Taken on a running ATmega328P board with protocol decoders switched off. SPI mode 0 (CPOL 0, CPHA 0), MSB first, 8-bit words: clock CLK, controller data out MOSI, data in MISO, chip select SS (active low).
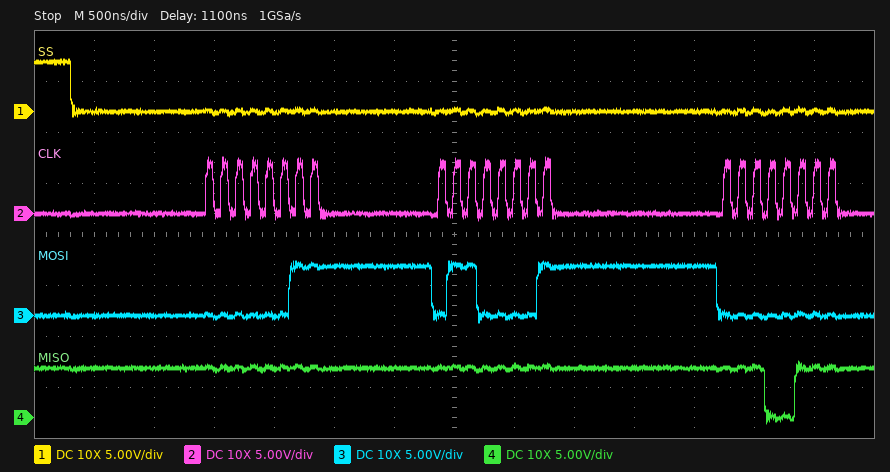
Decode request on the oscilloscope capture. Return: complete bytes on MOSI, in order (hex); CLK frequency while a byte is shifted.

03 61 00
8 MHz
